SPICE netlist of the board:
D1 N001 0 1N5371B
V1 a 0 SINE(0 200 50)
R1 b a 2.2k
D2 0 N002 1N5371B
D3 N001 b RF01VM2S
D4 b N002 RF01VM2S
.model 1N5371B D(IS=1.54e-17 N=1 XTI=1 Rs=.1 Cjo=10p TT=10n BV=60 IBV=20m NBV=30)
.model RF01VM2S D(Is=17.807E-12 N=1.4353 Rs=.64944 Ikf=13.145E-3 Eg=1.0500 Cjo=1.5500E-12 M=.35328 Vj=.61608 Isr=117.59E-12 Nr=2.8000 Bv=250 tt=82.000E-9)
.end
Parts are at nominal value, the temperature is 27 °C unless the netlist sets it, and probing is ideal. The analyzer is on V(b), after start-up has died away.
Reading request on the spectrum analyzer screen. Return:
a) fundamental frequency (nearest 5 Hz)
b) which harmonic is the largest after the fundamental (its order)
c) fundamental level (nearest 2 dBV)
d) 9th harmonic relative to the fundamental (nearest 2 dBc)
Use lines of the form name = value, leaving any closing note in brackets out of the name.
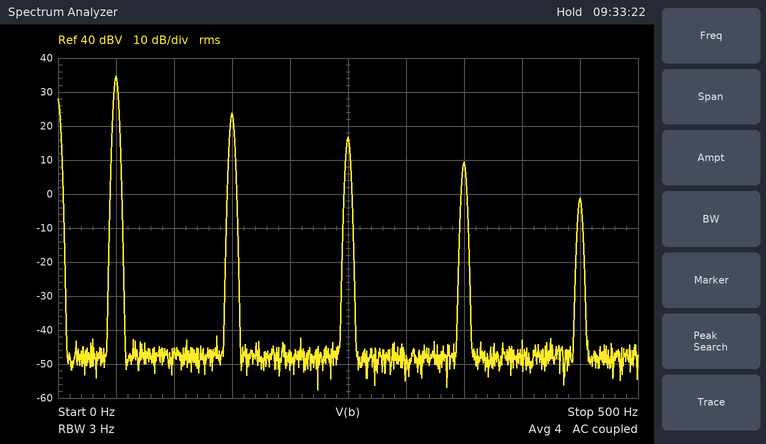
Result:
fundamental frequency = 50 Hz
which harmonic is the largest after the fundamental = 3
fundamental level = 34 dBV
9th harmonic relative to the fundamental = -36 dBc
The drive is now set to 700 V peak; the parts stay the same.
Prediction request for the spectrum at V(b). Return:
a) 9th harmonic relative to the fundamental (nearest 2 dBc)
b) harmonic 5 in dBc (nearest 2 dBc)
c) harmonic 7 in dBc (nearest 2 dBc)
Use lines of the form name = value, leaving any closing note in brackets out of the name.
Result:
9th harmonic relative to the fundamental = -20 dBc
harmonic 5 in dBc = -14 dBc
harmonic 7 in dBc = -18 dBc
